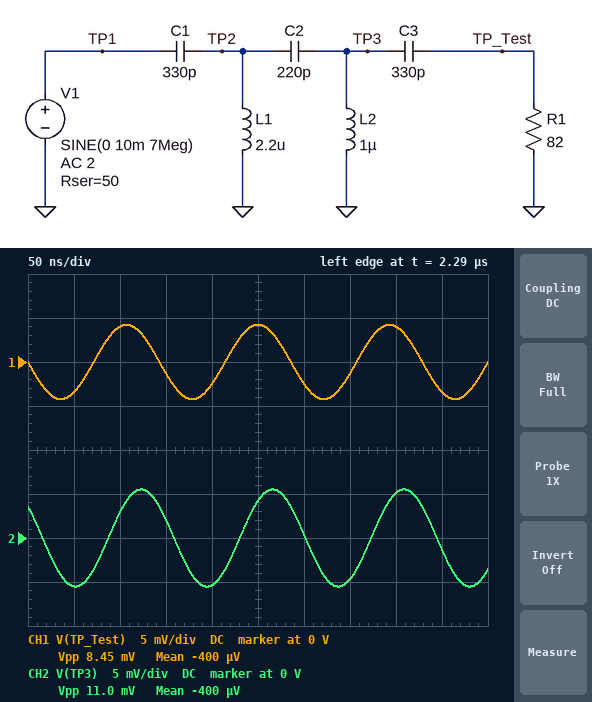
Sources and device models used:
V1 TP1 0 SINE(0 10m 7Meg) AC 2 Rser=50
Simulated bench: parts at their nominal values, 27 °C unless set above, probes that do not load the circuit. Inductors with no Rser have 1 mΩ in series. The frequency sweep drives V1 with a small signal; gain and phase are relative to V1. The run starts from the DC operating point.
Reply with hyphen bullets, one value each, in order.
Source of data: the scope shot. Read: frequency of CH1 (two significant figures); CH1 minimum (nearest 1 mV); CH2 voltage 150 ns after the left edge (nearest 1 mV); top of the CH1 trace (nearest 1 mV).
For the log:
- 7.0 MHz
- -4 mV
- 2 mV
- 4 mV
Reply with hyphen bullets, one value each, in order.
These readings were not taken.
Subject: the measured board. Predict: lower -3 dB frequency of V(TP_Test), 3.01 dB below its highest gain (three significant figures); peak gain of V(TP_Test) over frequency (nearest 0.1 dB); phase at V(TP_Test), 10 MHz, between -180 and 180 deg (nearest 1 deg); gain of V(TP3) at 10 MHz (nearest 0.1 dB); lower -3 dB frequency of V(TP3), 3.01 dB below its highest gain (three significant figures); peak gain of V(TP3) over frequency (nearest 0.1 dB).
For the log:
- 7.33 MHz
- -4.0 dB
- 126 deg
- -3.4 dB
- 4.34 MHz
- -3.3 dB
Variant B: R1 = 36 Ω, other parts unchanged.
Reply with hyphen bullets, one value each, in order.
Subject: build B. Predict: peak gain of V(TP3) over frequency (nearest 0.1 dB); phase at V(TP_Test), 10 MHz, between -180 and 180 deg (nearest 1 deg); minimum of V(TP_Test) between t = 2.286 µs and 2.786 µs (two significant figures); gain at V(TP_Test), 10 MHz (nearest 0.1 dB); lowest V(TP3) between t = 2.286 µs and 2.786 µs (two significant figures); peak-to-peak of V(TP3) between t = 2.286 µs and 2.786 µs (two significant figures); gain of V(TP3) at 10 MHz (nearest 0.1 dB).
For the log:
- -2.2 dB
- 118 deg
- -3.4 mV
- -8.1 dB
- -7.3 mV
- 15 mV
- -3.6 dB
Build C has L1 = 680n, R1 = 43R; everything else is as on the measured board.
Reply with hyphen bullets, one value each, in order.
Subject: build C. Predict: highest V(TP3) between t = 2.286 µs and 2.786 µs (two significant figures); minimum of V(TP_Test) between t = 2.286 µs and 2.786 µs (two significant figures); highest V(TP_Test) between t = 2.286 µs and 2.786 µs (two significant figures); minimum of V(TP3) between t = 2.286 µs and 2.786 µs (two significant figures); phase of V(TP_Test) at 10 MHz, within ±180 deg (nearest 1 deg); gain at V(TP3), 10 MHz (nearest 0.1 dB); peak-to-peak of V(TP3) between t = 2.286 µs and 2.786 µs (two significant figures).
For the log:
- 7.6 mV
- -4.0 mV
- 4.0 mV
- -7.6 mV
- 163 deg
- -3.9 dB
- 15 mV
